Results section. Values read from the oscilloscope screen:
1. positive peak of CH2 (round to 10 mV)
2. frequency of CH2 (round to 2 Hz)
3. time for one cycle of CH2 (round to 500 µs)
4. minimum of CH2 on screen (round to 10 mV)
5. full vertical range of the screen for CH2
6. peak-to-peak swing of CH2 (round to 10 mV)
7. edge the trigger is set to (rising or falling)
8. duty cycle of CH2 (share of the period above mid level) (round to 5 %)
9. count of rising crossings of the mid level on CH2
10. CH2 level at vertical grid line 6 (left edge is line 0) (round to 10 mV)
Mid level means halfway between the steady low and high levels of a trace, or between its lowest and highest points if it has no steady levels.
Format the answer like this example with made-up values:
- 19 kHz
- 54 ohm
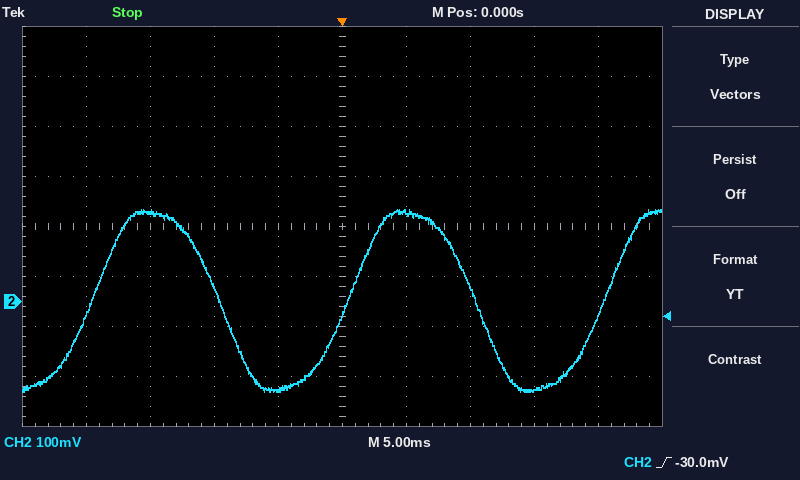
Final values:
- 180 mV
- 50 Hz
- 20.0 ms
- -180 mV
- 800 mV
- 360 mV
- rising
- 50 %
- 3
- 180 mV
